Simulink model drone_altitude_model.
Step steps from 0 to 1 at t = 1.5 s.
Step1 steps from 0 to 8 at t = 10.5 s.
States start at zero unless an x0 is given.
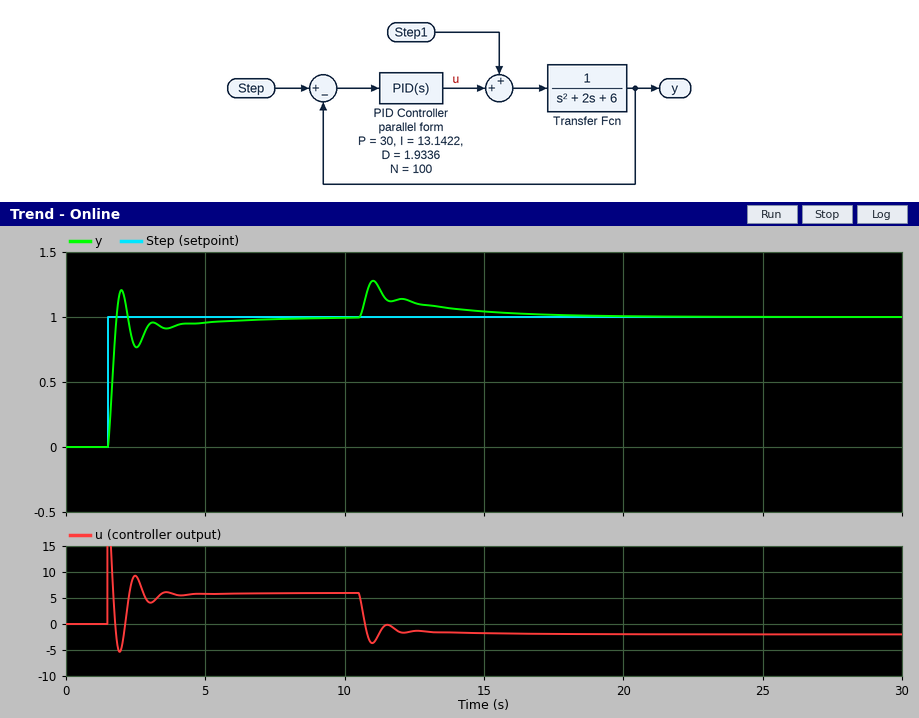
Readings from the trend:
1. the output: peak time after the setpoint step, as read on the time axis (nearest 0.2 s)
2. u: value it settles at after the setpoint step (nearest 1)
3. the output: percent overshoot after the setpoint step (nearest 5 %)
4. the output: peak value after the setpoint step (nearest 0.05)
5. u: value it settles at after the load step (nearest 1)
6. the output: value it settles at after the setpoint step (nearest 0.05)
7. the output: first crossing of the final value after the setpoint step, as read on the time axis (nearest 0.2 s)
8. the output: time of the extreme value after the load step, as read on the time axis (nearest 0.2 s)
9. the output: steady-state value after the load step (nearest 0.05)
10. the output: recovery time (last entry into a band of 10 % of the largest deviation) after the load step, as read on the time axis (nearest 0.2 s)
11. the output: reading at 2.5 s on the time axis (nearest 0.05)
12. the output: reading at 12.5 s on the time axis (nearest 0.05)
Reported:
2.0 s
6
20 %
1.20
-2
1.00
1.8 s
11.0 s
1.00
16.0 s
0.75
1.10
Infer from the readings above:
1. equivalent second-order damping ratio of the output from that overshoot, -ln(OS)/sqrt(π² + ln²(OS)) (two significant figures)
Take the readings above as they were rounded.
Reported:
0.46
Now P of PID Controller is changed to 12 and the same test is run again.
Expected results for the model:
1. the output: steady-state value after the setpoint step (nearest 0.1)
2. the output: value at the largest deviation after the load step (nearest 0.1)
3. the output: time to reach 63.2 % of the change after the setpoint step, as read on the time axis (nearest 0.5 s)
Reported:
1.0
1.5
2.0 s
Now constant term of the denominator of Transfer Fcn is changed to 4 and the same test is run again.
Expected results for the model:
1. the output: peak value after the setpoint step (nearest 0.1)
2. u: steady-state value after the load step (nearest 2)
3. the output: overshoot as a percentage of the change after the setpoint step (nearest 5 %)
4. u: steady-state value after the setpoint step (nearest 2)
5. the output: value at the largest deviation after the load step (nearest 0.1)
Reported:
1.3
-4
25 %
4
1.3
